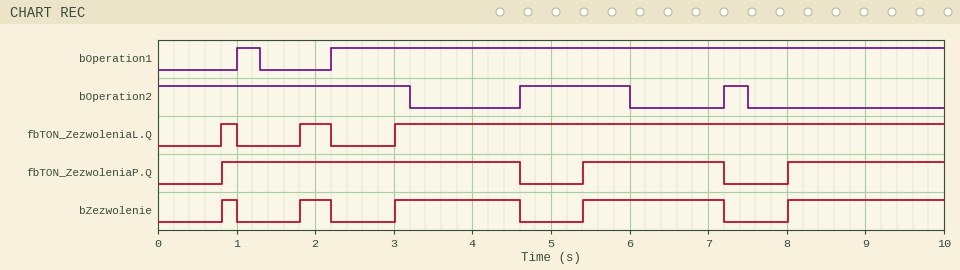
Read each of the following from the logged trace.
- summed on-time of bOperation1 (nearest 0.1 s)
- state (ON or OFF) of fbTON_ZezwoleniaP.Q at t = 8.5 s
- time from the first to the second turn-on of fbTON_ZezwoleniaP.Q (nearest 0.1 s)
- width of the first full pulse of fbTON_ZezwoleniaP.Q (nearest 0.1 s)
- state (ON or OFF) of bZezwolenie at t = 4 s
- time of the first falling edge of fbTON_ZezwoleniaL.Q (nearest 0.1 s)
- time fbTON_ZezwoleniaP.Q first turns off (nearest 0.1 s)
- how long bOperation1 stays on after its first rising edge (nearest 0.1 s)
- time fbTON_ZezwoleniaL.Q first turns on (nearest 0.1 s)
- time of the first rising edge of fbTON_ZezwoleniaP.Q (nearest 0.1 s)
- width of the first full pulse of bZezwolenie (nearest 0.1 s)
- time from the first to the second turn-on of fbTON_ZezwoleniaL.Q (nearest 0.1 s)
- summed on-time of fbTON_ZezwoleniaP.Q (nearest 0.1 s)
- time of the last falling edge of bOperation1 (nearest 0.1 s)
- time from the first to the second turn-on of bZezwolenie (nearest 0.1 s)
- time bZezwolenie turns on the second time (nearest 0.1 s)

8.1 s
ON
4.6 s
3.8 s
ON
1.0 s
4.6 s
0.3 s
0.8 s
0.8 s
0.2 s
1.0 s
7.6 s
1.3 s
1.0 s
1.8 s
